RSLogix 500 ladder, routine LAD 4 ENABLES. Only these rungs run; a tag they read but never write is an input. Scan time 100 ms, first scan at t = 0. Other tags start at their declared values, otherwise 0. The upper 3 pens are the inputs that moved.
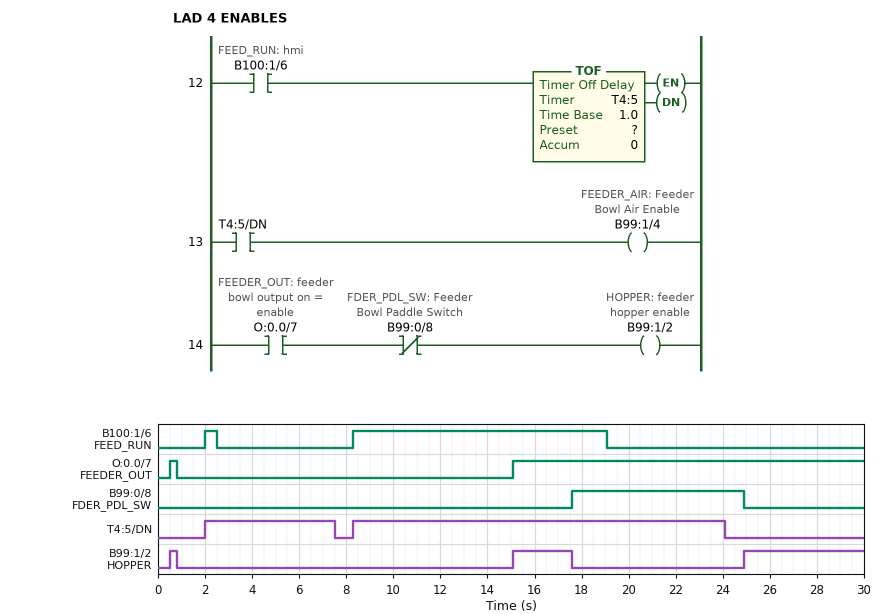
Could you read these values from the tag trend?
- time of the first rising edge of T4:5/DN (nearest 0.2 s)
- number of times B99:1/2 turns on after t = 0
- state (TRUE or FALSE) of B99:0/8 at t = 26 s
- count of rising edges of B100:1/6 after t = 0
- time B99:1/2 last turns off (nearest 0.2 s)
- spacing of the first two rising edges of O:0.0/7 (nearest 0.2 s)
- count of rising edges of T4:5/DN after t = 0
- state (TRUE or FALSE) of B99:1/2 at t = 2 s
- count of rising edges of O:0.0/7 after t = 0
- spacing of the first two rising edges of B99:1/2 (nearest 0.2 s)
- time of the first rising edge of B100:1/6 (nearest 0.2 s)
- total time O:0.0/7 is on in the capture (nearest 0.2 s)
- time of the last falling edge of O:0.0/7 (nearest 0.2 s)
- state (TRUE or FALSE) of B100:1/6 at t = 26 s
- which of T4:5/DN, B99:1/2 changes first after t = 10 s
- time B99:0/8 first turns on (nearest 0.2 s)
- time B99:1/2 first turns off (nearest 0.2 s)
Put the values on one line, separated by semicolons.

2.0 s; 3; FALSE; 2; 17.6 s; 14.6 s; 2; FALSE; 2; 14.6 s; 2.0 s; 15.2 s; 0.8 s; FALSE; B99:1/2; 17.6 s; 0.8 s
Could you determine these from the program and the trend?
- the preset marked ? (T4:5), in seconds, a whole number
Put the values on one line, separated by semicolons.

5 s
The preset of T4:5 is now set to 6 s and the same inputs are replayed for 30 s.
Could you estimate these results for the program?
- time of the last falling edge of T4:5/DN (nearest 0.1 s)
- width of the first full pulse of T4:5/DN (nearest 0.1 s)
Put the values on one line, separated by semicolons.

25.1 s; 23.1 s
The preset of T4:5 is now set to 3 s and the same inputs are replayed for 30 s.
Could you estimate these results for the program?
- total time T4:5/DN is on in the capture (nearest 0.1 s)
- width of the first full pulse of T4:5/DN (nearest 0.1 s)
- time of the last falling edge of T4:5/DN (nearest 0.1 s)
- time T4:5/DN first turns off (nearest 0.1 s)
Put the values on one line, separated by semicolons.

17.3 s; 3.5 s; 22.1 s; 5.5 s
